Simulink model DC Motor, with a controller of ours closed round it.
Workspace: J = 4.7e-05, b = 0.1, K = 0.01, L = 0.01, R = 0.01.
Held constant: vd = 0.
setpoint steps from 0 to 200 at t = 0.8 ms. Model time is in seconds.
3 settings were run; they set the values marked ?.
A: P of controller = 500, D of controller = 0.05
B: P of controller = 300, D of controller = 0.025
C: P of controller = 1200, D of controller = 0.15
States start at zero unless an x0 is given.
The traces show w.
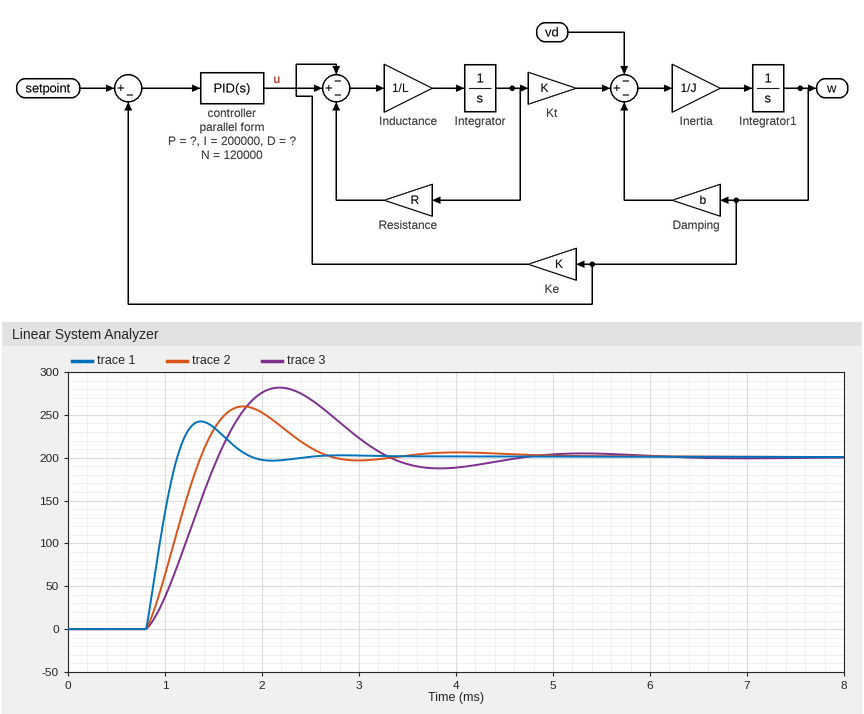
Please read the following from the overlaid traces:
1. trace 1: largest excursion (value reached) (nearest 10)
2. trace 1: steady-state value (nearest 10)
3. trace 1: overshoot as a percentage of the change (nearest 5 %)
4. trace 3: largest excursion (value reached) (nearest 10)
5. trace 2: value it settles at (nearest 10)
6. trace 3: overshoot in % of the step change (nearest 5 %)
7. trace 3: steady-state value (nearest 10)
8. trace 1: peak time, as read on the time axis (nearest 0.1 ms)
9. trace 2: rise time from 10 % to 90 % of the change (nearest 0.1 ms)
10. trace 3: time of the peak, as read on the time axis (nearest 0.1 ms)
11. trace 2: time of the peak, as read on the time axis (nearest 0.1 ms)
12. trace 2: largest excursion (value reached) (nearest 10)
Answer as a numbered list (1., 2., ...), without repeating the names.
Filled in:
1. 240
2. 200
3. 20 %
4. 280
5. 200
6. 40 %
7. 200
8. 1.4 ms
9. 0.4 ms
10. 2.2 ms
11. 1.8 ms
12. 260
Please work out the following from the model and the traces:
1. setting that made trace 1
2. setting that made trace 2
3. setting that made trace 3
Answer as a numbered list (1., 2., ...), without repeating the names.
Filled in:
1. C
2. A
3. B
